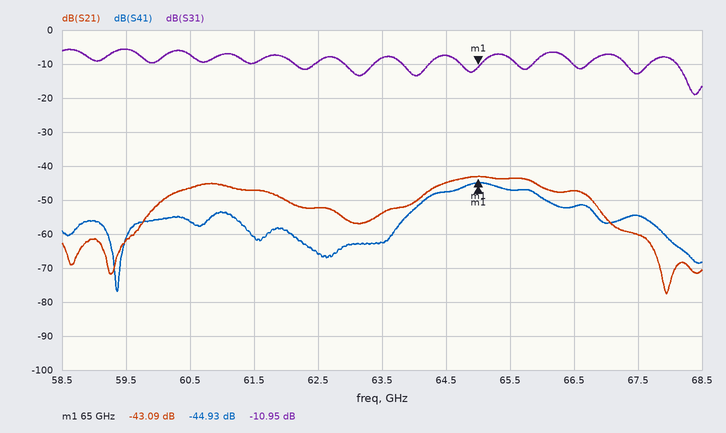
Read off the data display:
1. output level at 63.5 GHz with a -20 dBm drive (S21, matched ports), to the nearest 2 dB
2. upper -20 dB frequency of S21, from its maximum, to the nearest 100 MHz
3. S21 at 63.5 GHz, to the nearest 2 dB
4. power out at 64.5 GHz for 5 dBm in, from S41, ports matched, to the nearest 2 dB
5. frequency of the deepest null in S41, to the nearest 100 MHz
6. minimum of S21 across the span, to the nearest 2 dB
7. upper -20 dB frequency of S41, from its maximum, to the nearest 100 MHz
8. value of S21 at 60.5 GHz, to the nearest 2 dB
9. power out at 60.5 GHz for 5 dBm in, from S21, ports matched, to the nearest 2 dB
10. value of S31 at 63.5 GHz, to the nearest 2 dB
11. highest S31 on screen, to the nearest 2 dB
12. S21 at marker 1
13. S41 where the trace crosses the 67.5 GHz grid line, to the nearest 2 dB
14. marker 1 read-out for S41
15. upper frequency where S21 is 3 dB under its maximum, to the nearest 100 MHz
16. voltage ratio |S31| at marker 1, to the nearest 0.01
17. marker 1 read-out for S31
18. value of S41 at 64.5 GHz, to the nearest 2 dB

-74 dBm
67.7 GHz
-54 dB
-42 dBm
59.4 GHz
-78 dB
68.2 GHz
-46 dB
-42 dBm
-8 dB
-6 dB
-43.09 dB
-54 dB
-44.93 dB
66.0 GHz
0.28
-10.95 dB
-48 dB
